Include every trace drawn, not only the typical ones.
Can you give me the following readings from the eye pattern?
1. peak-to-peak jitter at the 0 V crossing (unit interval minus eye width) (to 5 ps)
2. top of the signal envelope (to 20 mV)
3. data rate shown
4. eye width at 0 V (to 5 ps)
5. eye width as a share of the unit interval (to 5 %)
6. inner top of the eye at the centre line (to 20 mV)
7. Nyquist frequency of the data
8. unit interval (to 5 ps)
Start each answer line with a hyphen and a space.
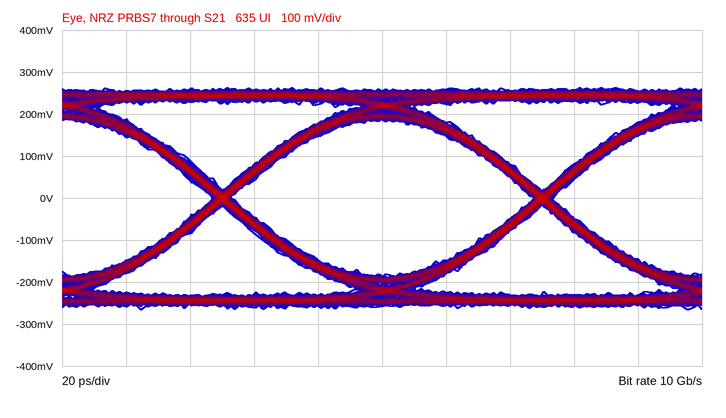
- 5 ps
- 260 mV
- 10 Gb/s
- 95 ps
- 95 %
- 180 mV
- 5 GHz
- 100 ps
